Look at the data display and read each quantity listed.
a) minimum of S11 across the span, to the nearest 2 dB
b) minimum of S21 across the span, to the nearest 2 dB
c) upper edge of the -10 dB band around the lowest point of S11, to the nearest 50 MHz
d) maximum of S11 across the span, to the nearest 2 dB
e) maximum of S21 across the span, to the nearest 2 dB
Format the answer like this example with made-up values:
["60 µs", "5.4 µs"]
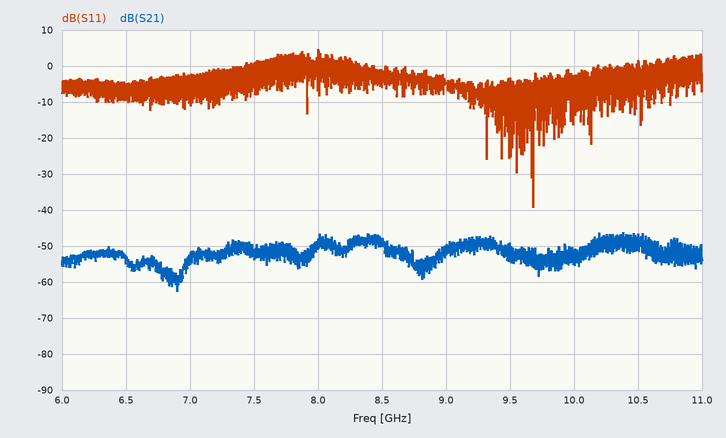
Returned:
["-40 dB", "-62 dB", "9.70 GHz", "4 dB", "-46 dB"]
